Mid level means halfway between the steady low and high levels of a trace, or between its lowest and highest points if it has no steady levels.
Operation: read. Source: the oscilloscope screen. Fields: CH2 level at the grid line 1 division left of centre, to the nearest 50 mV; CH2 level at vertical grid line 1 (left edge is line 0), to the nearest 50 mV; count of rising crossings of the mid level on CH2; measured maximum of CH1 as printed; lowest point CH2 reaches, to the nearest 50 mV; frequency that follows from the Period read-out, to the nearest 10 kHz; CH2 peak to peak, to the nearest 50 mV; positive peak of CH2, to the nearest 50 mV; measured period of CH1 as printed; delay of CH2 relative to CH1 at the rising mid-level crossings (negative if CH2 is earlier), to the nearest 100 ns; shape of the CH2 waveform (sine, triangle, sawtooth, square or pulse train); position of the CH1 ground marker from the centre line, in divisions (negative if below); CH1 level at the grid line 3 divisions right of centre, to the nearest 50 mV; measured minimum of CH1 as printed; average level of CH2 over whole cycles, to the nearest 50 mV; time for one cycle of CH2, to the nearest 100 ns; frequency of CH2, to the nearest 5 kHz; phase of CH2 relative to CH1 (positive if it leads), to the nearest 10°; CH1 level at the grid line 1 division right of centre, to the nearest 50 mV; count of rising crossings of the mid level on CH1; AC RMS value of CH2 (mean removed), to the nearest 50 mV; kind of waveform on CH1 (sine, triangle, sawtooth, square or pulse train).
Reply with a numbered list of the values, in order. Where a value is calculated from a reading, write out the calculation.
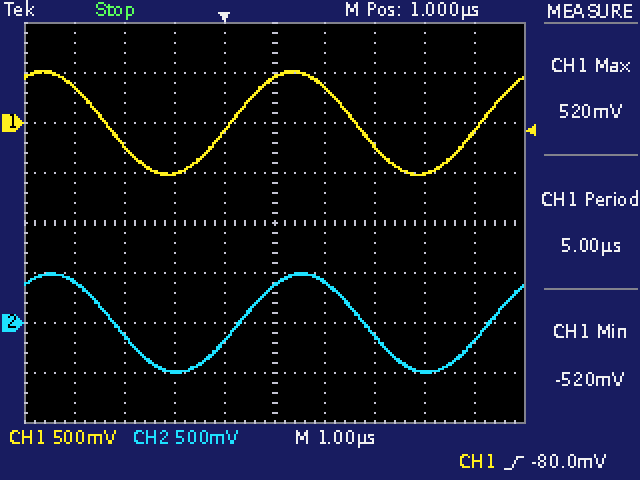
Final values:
1. -200 mV
2. 400 mV
3. 2
4. 520 mV
5. -500 mV
6. 1 / 5.00 µs ≈ 200 kHz
7. 500 mV − (-500 mV) = 1.00 V
8. 500 mV
9. 5.00 µs
10. +200 ns
11. sine
12. +2.0 div
13. -500 mV
14. -520 mV
15. (500 mV + (-500 mV)) / 2 ≈ 0 mV
16. 5.0 µs
17. 1 / 5.0 µs ≈ 200 kHz
18. −360° × (+200 ns) / 5.0 µs ≈ -14.4°, so -10° to the nearest 10°
19. 350 mV
20. 2
21. 1.00 V / (2√2) ≈ 354 mV, so 350 mV to the nearest 50 mV
22. sine
